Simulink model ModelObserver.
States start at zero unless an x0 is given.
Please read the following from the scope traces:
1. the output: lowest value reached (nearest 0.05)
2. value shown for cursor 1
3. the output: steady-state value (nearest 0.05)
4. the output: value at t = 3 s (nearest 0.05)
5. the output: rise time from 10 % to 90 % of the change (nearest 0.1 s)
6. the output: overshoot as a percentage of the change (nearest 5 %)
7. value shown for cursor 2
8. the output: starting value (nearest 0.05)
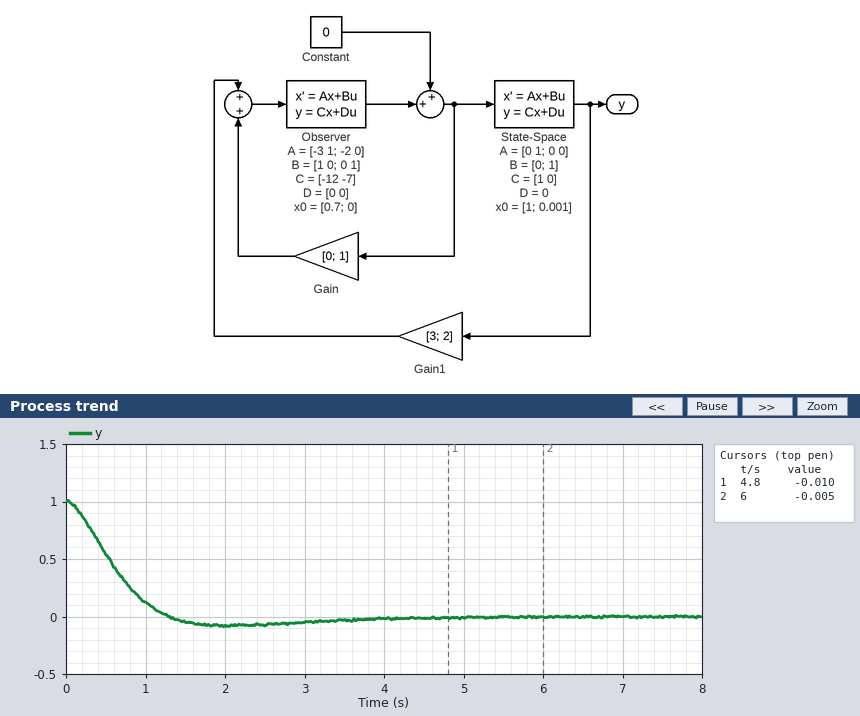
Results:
-0.10
-0.010
0.00
-0.05
0.9 s
10 %
-0.005
1.00
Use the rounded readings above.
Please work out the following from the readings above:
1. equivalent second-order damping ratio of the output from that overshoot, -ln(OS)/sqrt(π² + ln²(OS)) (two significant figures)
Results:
0.59
